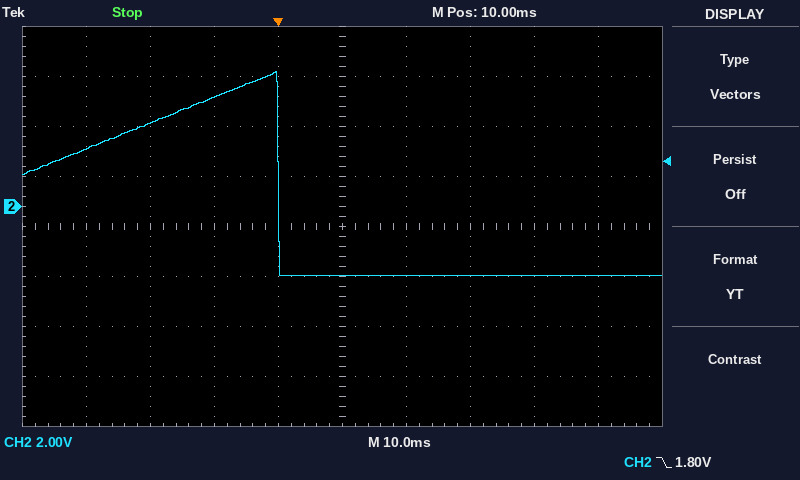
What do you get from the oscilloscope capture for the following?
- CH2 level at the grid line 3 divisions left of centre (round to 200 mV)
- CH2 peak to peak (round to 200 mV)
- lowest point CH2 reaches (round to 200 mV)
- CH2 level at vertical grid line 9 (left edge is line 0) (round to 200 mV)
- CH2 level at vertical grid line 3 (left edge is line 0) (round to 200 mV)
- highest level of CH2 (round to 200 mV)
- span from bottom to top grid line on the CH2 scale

3.4 V
8.2 V
-2.8 V
-2.8 V
4.4 V
5.4 V
16 V
